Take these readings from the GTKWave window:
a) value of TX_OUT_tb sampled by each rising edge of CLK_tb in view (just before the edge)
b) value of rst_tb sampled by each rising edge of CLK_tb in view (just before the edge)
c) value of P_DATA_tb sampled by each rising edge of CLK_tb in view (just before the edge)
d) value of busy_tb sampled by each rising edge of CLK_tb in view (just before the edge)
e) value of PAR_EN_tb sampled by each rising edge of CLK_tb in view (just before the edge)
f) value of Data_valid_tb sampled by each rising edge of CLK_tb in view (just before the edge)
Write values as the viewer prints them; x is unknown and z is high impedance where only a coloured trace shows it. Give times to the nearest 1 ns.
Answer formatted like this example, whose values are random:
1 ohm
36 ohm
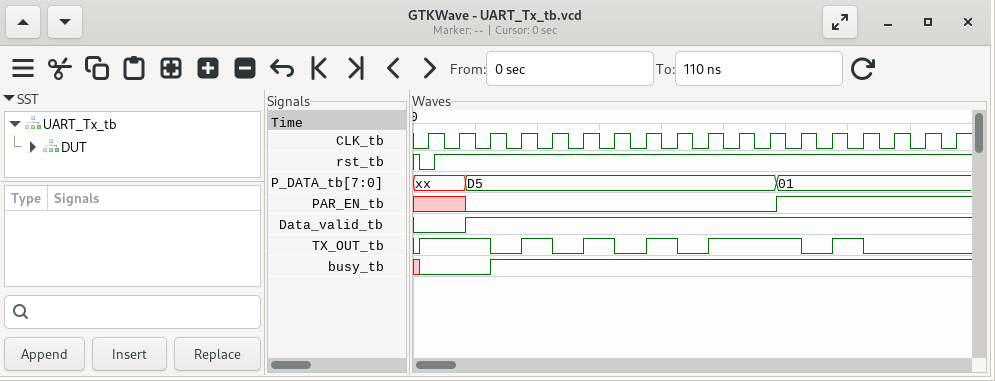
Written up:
1 1 1 0 1 0 1 0 1 0 1 1 1 0 1 0 0 0
0 1 1 1 1 1 1 1 1 1 1 1 1 1 1 1 1 1
xx, xx, D5, D5, D5, D5, D5, D5, D5, D5, D5, D5, 01, 01, 01, 01, 01, 01
0 0 0 1 1 1 1 1 1 1 1 1 1 1 1 1 1 1
x x 0 0 0 0 0 0 0 0 0 0 1 1 1 1 1 1
0 0 1 1 1 1 1 1 1 1 1 1 1 1 1 1 1 1
